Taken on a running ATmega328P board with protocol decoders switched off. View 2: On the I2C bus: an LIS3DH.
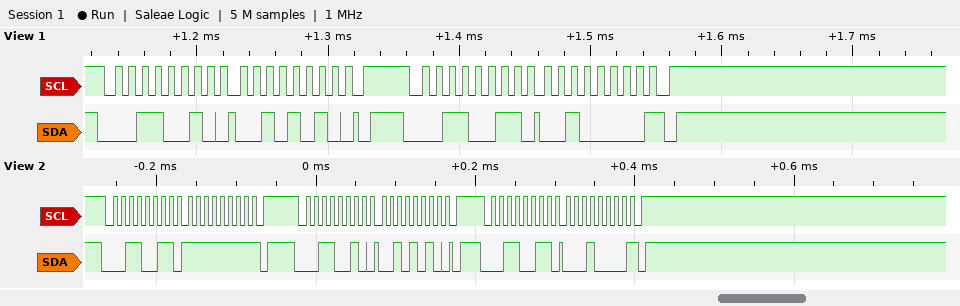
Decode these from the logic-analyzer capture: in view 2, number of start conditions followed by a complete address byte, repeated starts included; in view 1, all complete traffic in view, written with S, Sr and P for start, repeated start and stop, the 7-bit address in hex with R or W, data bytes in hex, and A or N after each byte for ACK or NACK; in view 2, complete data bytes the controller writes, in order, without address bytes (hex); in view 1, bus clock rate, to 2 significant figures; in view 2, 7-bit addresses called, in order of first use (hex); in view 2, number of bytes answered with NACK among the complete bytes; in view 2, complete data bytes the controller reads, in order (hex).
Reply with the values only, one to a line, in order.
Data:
3
S 19W A 2A A P S 19R A 20 N P
2A
100 kHz
0x19
2
FF 10
